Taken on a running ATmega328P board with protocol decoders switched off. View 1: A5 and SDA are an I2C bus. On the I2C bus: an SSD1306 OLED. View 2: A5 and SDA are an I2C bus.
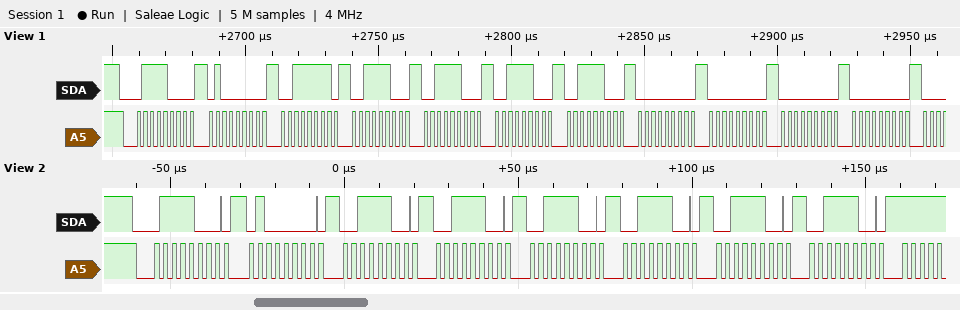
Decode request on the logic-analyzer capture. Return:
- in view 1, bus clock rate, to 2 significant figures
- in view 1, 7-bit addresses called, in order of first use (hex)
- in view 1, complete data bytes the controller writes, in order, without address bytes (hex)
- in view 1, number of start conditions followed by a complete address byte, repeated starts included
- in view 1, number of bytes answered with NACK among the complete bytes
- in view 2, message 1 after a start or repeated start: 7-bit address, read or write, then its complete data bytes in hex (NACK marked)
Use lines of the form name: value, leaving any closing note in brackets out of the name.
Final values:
in view 1, bus clock rate, to 2 significant figures: 400 kHz
in view 1, 7-bit addresses called, in order of first use: 0x3C
in view 1, complete data bytes the controller writes, in order, without address bytes: 40 3F 3C 3C 3C 3C 00 00 00 00
in view 1, number of start conditions followed by a complete address byte, repeated starts included: 1
in view 1, number of bytes answered with NACK among the complete bytes: 0
in view 2, message 1 after a start or repeated start: 7-bit address, read or write, then its complete data bytes in hex: 0x3C write: 40 3C 3C 3C 3C 3C 3C
